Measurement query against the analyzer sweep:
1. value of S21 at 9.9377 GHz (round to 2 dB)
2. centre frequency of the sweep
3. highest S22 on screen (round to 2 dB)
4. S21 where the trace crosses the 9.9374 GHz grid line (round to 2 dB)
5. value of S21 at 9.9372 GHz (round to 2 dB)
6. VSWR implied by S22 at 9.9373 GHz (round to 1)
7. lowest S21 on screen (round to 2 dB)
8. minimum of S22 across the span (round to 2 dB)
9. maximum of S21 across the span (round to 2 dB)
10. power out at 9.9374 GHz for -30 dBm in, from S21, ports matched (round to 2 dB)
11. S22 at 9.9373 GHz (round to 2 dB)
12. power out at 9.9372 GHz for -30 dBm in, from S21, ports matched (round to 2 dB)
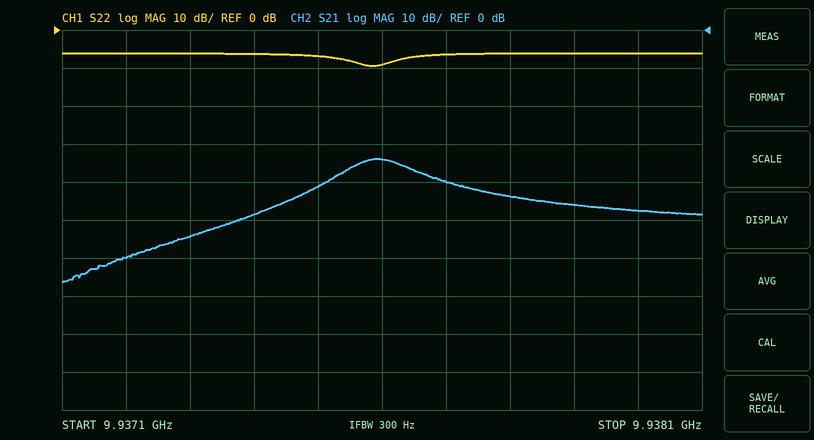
-40 dB
9.9376 GHz
-6 dB
-48 dB
-60 dB
3
-66 dB
-10 dB
-34 dB
-78 dBm
-6 dB
-90 dBm
